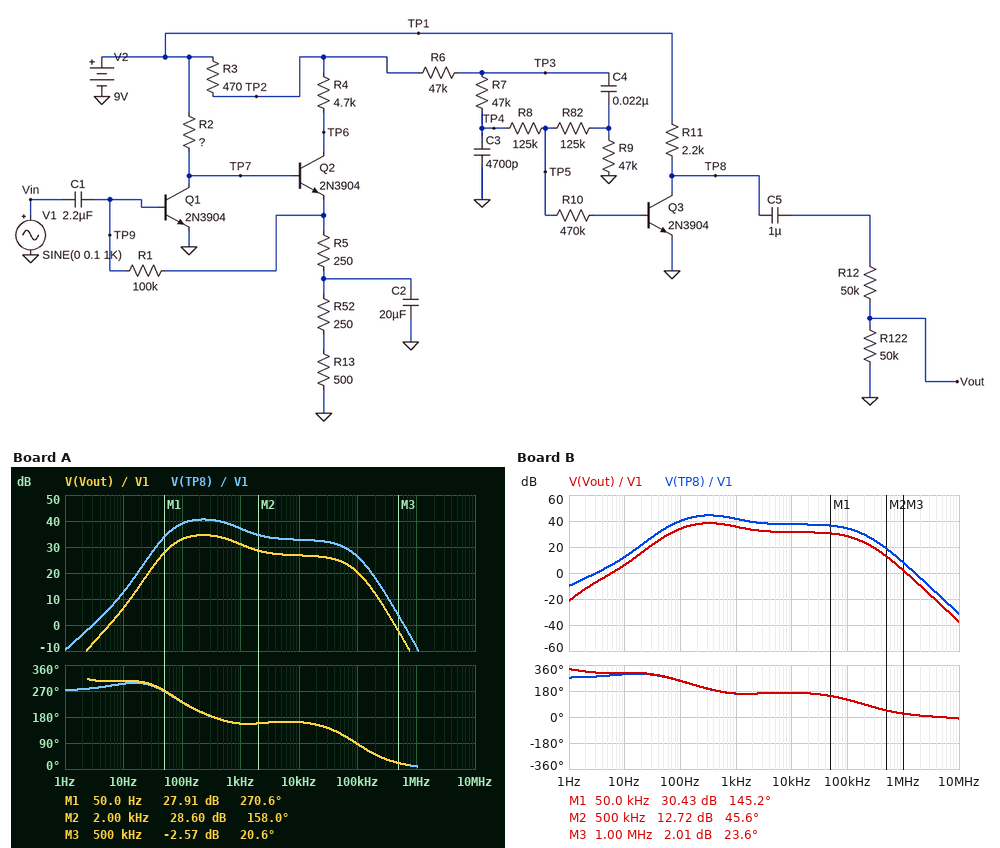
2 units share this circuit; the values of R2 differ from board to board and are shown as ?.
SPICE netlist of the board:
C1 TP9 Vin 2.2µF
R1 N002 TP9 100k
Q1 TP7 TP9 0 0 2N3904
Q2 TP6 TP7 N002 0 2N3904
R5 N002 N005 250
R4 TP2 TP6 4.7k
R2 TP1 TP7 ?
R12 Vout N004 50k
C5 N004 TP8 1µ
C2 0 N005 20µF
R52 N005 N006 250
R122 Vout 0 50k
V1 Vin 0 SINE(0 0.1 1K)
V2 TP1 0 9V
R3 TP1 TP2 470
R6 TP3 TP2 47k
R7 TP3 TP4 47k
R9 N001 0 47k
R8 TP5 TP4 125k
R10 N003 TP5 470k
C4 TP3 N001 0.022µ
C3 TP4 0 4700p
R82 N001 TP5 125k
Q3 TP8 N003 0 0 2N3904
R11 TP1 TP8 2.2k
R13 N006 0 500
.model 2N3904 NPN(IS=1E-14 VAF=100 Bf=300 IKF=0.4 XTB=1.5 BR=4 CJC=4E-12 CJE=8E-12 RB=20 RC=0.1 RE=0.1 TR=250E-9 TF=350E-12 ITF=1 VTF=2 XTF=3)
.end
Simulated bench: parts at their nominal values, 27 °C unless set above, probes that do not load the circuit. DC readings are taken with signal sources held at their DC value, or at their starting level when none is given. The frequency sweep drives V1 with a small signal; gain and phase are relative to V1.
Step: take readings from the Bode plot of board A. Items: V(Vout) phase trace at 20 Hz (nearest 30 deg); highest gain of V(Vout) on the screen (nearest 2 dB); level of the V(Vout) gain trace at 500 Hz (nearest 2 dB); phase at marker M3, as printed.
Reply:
300 deg
34 dB
34 dB
20.6 deg
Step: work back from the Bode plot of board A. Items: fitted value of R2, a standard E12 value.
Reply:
82 kΩ
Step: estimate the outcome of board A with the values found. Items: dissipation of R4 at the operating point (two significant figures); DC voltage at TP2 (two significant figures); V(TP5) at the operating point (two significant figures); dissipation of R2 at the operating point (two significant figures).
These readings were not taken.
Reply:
1.8 mW
8.7 V
3.3 V
730 µW
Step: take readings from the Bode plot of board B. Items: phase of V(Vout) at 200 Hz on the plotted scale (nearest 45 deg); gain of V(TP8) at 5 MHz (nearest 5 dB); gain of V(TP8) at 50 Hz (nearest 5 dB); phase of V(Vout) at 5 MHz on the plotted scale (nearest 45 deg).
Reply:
225 deg
-20 dB
35 dB
0 deg
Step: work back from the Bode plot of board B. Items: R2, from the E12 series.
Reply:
10 kΩ
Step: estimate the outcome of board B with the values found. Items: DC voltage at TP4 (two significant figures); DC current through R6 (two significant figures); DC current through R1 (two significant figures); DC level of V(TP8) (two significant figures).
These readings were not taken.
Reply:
6.3 V
24 µA
2.5 µA
5.2 V
